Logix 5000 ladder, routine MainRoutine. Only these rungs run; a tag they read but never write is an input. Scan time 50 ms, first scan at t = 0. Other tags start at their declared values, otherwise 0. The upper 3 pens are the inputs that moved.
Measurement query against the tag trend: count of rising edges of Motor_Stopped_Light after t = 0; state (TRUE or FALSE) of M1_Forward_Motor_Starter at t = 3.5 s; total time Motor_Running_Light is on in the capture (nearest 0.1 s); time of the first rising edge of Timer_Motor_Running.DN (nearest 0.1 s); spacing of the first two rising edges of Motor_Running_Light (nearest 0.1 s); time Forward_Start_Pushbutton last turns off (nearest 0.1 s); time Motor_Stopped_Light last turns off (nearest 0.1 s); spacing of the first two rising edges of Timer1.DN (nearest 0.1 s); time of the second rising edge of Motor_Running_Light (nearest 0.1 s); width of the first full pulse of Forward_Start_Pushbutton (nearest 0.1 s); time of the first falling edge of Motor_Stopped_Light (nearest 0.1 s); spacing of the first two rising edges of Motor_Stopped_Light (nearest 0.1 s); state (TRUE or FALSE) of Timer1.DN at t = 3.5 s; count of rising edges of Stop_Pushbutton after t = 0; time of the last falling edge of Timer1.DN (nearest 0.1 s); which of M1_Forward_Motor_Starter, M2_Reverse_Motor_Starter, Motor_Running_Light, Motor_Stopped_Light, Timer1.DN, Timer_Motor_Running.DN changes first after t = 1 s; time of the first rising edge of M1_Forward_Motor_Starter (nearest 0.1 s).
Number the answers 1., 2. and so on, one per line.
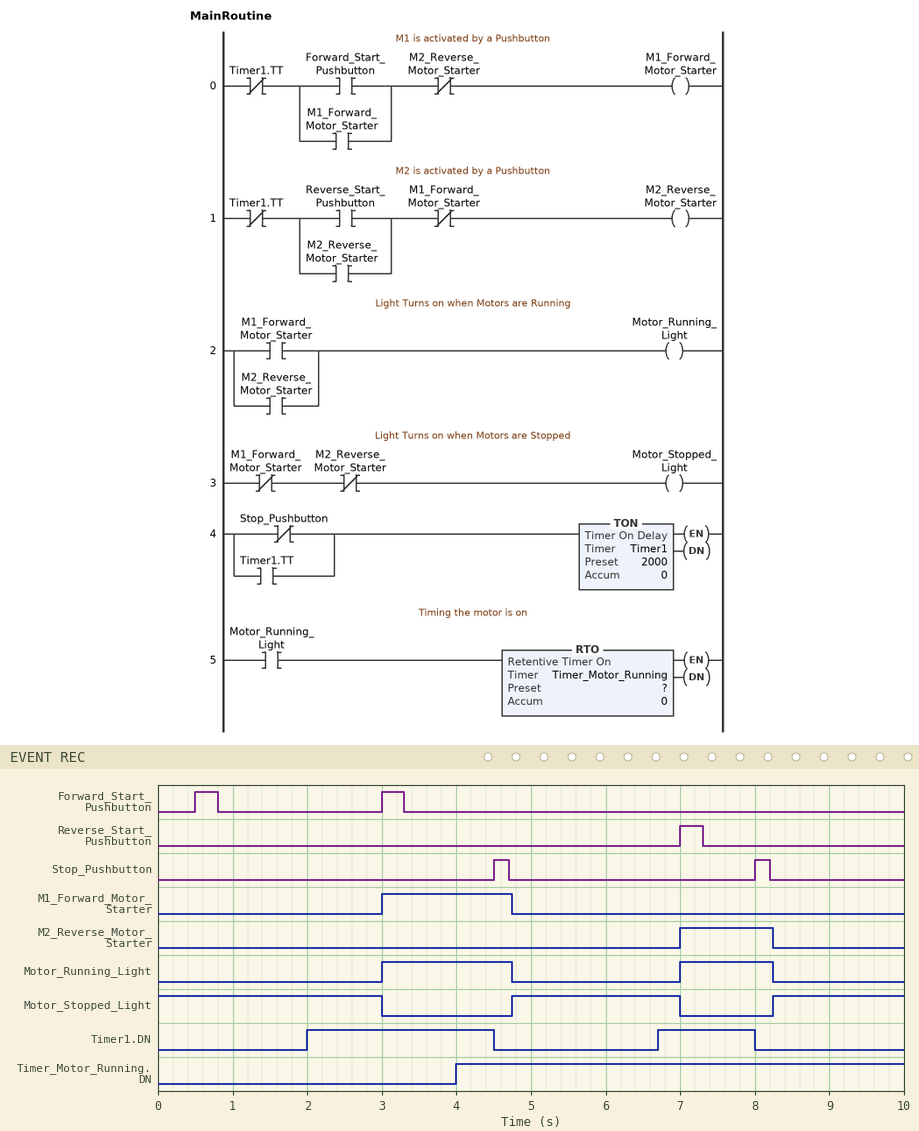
1. 2
2. TRUE
3. 3.0 s
4. 4.0 s
5. 4.0 s
6. 3.3 s
7. 7.0 s
8. 4.7 s
9. 7.0 s
10. 0.3 s
11. 3.0 s
12. 3.5 s
13. TRUE
14. 2
15. 8.0 s
16. Timer1.DN
17. 3.0 s
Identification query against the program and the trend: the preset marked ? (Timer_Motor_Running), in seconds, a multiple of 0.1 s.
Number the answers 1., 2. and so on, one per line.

1. 1.0 s
